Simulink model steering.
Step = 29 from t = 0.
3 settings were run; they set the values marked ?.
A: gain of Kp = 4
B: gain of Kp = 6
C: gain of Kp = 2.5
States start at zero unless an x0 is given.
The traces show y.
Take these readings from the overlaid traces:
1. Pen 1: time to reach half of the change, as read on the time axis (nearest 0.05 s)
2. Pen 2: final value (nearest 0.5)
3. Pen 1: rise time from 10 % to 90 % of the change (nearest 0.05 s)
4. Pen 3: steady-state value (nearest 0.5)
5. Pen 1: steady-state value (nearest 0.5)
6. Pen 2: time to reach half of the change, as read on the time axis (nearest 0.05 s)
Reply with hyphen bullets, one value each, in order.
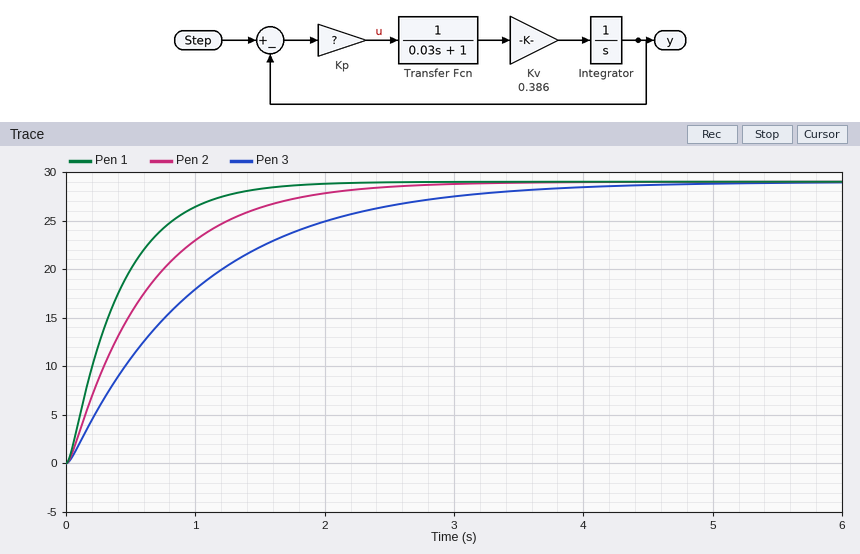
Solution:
- 0.30 s
- 29.0
- 0.90 s
- 29.0
- 29.0
- 0.45 s
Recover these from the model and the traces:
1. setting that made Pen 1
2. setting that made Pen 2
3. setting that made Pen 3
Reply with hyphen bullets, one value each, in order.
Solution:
- B
- A
- C
